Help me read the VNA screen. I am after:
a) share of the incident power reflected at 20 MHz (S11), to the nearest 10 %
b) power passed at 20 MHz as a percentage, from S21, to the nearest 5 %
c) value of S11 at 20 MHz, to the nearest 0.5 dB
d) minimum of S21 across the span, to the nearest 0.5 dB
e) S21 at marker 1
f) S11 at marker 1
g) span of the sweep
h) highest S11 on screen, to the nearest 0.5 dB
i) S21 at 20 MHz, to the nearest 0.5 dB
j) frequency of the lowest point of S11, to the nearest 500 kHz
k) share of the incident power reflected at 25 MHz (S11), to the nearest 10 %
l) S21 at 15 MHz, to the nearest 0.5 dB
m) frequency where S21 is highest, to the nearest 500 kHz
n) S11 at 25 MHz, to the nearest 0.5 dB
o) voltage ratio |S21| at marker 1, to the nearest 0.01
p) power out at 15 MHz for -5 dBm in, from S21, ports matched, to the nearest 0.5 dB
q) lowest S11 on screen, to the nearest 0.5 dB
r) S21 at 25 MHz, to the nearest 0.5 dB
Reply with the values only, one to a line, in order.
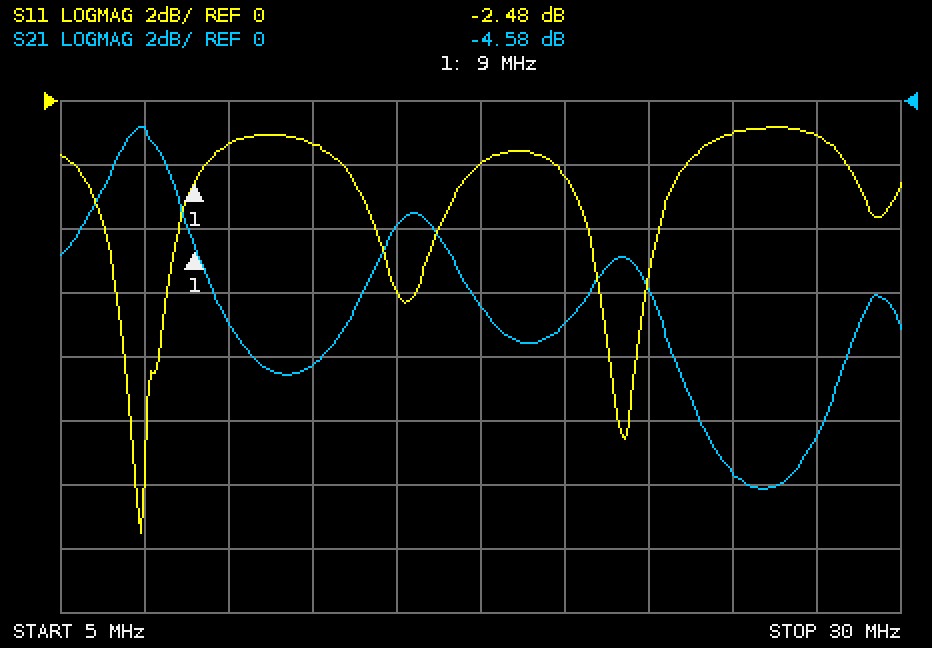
60 %
20 %
-2.5 dB
-12.0 dB
-4.58 dB
-2.48 dB
25 MHz
-1.0 dB
-7.0 dB
7.5 MHz
80 %
-4.0 dB
7.5 MHz
-1.0 dB
0.59
-9.0 dBm
-13.5 dB
-11.5 dB
